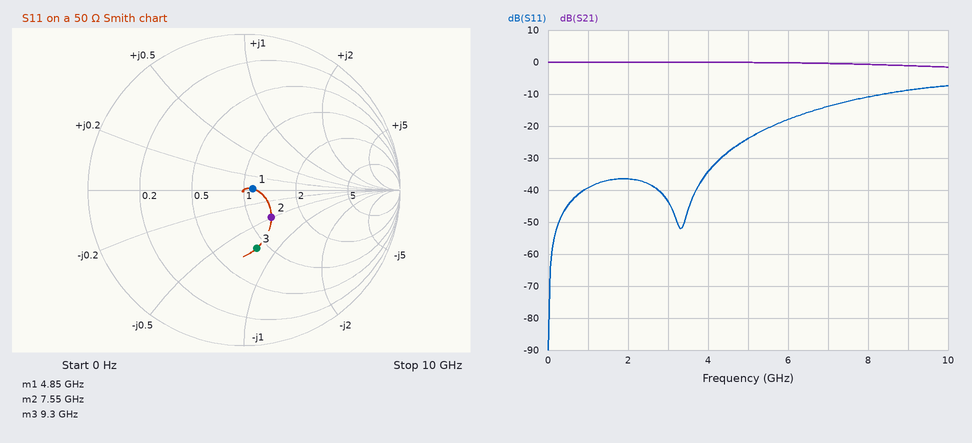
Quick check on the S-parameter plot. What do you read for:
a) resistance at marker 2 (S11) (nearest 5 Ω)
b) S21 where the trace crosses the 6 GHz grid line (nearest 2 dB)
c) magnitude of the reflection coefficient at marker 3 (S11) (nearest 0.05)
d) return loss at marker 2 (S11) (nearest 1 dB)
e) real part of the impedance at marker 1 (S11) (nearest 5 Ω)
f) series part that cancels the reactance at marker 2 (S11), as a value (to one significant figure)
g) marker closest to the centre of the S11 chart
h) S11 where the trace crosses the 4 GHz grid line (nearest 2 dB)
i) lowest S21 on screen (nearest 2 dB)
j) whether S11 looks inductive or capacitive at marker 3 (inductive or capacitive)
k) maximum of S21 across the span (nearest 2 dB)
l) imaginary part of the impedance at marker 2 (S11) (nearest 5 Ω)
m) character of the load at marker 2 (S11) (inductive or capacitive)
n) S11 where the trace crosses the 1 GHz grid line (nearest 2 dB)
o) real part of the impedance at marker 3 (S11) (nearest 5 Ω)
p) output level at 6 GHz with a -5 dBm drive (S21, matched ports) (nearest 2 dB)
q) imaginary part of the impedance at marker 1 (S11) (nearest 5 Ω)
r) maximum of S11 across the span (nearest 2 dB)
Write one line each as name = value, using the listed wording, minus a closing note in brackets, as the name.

resistance at marker 2 (S11) = 65 Ω
S21 where the trace crosses the 6 GHz grid line = 0 dB
magnitude of the reflection coefficient at marker 3 (S11) = 0.40
return loss at marker 2 (S11) = 12 dB
real part of the impedance at marker 1 (S11) = 55 Ω
series part that cancels the reactance at marker 2 (S11), as a value = 500 pH
marker closest to the centre of the S11 chart = marker 1
S11 where the trace crosses the 4 GHz grid line = -34 dB
lowest S21 on screen = -2 dB
whether S11 looks inductive or capacitive at marker 3 = capacitive
maximum of S21 across the span = 0 dB
imaginary part of the impedance at marker 2 (S11) = -25 Ω
character of the load at marker 2 (S11) = capacitive
S11 where the trace crosses the 1 GHz grid line = -40 dB
real part of the impedance at marker 3 (S11) = 45 Ω
output level at 6 GHz with a -5 dBm drive (S21, matched ports) = -6 dBm
imaginary part of the impedance at marker 1 (S11) = 0 Ω
maximum of S11 across the span = -8 dB
